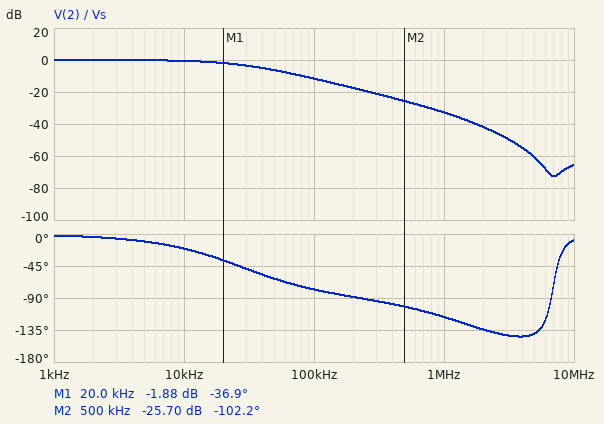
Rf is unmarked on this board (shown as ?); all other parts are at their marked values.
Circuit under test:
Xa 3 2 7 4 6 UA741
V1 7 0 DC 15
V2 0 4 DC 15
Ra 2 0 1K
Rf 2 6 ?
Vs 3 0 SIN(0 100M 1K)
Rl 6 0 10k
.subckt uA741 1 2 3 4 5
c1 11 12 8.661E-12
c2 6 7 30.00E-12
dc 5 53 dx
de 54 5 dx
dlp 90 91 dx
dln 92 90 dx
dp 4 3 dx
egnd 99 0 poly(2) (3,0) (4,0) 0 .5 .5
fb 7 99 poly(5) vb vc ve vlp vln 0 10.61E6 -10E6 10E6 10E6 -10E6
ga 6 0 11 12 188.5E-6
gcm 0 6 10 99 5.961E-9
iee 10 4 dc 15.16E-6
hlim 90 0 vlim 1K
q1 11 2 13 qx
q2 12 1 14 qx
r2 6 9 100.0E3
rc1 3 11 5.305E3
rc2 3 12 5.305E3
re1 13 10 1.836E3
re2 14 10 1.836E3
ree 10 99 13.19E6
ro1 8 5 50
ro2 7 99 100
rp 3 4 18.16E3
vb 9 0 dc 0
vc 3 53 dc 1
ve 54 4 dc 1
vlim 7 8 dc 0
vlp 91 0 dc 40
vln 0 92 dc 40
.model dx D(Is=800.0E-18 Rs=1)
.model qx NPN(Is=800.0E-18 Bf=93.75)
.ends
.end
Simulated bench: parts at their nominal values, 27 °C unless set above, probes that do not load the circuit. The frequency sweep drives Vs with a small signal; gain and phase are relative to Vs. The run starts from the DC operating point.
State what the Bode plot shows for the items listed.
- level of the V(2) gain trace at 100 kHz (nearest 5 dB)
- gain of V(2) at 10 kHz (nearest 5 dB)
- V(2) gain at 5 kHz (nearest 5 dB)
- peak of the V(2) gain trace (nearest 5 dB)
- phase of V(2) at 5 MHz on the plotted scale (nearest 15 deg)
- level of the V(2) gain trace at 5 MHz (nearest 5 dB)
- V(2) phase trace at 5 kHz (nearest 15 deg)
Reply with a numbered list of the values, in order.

1. -10 dB
2. 0 dB
3. 0 dB
4. 0 dB
5. -135 deg
6. -60 dB
7. -15 deg
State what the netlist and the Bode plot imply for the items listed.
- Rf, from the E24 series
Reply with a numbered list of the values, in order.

1. 36 kΩ
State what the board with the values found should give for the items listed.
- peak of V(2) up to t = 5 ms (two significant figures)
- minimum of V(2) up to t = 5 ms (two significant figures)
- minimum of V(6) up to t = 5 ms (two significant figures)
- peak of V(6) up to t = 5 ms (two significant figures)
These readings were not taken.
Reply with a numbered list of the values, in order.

1. 100 mV
2. -100 mV
3. -3.7 V
4. 3.7 V
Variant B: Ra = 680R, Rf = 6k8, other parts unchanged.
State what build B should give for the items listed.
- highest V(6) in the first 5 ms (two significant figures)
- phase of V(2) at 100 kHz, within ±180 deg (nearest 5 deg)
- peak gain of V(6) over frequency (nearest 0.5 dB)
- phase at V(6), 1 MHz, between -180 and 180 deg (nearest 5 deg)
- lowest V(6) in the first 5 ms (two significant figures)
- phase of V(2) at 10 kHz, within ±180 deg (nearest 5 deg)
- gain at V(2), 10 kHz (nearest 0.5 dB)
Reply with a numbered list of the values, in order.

1. 1.1 V
2. -50 deg
3. 21.0 dB
4. -115 deg
5. -1.1 V
6. -5 deg
7. 0 dB
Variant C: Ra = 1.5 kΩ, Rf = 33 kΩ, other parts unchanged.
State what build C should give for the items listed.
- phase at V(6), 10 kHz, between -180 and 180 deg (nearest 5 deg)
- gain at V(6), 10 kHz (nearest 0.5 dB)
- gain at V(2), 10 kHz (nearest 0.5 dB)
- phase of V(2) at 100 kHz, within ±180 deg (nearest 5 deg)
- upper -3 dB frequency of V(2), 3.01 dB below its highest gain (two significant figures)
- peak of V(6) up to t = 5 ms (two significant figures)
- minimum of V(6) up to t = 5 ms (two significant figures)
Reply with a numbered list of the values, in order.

1. -15 deg
2. 27.0 dB
3. 0 dB
4. -70 deg
5. 44 kHz
6. 2.3 V
7. -2.3 V
